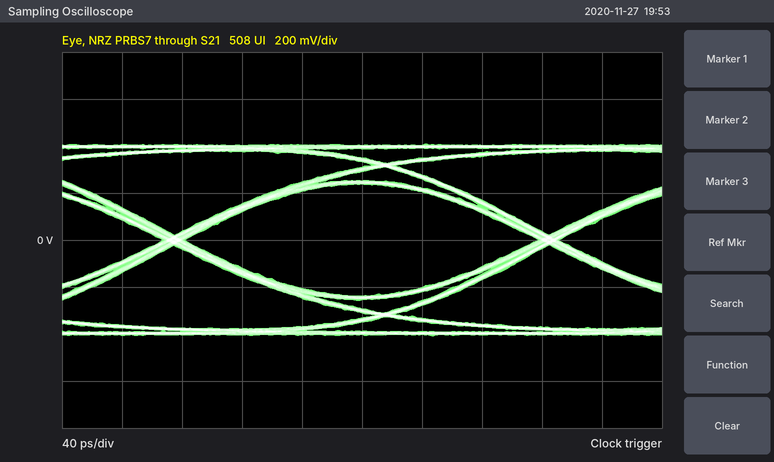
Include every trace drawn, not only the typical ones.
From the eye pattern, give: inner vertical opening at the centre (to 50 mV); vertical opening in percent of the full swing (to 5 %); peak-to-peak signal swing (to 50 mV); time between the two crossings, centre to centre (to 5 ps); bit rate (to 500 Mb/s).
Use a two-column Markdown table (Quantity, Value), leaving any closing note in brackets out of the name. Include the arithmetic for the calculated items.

| Quantity | Value |
|---|---|
| inner vertical opening at the centre | 500 mV |
| vertical opening in percent of the full swing | 500 mV / 800 mV ≈ 62.5 %, so 60 % to the nearest 5 % |
| peak-to-peak signal swing | 800 mV |
| time between the two crossings, centre to centre | 250 ps |
| bit rate | 4.0 Gb/s |
